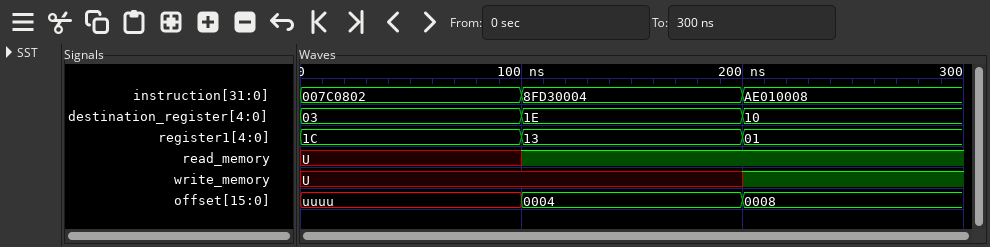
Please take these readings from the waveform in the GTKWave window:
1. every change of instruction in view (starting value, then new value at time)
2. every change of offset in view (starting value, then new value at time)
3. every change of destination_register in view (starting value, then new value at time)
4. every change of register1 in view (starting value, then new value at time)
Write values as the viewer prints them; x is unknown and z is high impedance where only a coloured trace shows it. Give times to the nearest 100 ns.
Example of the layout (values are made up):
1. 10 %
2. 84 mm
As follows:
1. 007C0802, 8FD30004 at 100 ns, AE010008 at 200 ns
2. uuuu, 0004 at 100 ns, 0008 at 200 ns
3. 03, 1E at 100 ns, 10 at 200 ns
4. 1C, 13 at 100 ns, 01 at 200 ns
